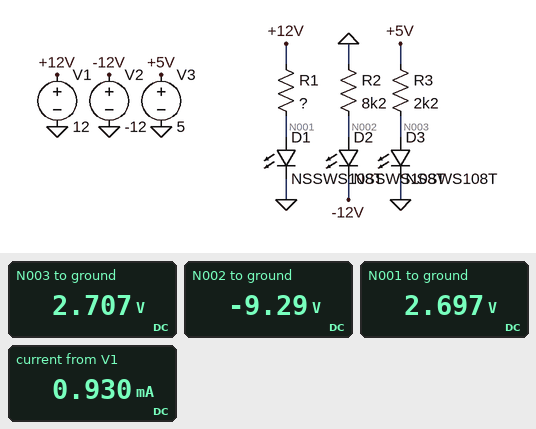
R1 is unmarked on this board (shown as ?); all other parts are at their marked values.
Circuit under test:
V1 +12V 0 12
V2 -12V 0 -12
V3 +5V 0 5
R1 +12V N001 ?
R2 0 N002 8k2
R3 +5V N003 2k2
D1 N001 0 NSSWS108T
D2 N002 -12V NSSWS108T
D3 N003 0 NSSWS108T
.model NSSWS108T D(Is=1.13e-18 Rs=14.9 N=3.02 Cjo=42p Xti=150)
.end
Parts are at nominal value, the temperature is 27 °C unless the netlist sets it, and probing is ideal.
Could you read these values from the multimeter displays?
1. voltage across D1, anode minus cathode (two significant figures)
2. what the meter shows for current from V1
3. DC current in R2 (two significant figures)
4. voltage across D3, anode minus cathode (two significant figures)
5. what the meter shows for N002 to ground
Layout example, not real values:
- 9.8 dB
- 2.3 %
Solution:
- 2.7 V
- 0.930 mA
- 1.1 mA
- 2.7 V
- -9.29 V
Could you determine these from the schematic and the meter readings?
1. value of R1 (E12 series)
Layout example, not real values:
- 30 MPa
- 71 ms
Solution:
- 10 kΩ
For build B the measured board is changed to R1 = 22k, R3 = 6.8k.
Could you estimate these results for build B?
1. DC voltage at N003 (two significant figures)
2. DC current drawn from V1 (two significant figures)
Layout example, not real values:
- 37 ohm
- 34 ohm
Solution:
- 2.6 V
- 430 µA
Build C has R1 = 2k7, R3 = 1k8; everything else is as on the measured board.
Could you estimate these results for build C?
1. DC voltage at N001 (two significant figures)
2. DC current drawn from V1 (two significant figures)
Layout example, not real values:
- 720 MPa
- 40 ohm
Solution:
- 2.8 V
- 3.4 mA
